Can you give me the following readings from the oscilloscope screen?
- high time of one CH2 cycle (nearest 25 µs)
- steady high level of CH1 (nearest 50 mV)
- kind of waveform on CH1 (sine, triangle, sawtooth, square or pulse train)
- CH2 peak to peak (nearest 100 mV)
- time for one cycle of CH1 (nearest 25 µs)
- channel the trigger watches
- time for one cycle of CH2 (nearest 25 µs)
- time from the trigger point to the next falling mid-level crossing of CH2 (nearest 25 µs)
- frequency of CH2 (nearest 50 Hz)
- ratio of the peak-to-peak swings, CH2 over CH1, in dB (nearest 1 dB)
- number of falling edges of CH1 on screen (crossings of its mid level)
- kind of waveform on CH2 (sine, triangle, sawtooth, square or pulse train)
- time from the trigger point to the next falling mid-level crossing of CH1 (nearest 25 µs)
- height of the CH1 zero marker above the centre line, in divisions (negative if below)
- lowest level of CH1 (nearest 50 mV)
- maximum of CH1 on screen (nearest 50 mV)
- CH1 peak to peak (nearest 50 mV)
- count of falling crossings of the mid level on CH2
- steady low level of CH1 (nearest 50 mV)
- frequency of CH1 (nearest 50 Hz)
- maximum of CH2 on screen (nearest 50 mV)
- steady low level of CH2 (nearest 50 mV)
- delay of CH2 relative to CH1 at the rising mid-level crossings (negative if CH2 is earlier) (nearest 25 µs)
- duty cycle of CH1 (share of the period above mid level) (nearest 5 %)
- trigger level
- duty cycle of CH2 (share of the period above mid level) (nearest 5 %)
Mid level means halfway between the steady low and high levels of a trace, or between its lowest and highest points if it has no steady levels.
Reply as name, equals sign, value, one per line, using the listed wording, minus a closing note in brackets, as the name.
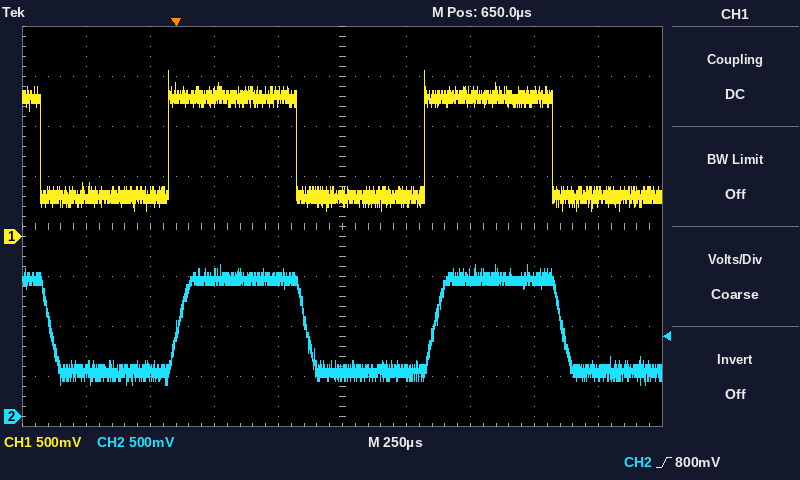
high time of one CH2 cycle = 500 µs
steady high level of CH1 = 1.40 V
kind of waveform on CH1 = square
CH2 peak to peak = 1.20 V
time for one cycle of CH1 = 1.000 ms
channel the trigger watches = CH2
time for one cycle of CH2 = 1.000 ms
time from the trigger point to the next falling mid-level crossing of CH2 = 500 µs
frequency of CH2 = 1.00 kHz
ratio of the peak-to-peak swings, CH2 over CH1, in dB = -1 dB
number of falling edges of CH1 on screen = 3
kind of waveform on CH2 = square
time from the trigger point to the next falling mid-level crossing of CH1 = 475 µs
height of the CH1 zero marker above the centre line, in divisions = -0.2 div
lowest level of CH1 = 250 mV
maximum of CH1 on screen = 1.65 V
CH1 peak to peak = 1.40 V
count of falling crossings of the mid level on CH2 = 3
steady low level of CH1 = 400 mV
frequency of CH1 = 1.00 kHz
maximum of CH2 on screen = 1.50 V
steady low level of CH2 = 450 mV
delay of CH2 relative to CH1 at the rising mid-level crossings (negative if CH2 is earlier) = +50 µs
duty cycle of CH1 (share of the period above mid level) = 50 %
trigger level = 800 mV
duty cycle of CH2 (share of the period above mid level) = 50 %
